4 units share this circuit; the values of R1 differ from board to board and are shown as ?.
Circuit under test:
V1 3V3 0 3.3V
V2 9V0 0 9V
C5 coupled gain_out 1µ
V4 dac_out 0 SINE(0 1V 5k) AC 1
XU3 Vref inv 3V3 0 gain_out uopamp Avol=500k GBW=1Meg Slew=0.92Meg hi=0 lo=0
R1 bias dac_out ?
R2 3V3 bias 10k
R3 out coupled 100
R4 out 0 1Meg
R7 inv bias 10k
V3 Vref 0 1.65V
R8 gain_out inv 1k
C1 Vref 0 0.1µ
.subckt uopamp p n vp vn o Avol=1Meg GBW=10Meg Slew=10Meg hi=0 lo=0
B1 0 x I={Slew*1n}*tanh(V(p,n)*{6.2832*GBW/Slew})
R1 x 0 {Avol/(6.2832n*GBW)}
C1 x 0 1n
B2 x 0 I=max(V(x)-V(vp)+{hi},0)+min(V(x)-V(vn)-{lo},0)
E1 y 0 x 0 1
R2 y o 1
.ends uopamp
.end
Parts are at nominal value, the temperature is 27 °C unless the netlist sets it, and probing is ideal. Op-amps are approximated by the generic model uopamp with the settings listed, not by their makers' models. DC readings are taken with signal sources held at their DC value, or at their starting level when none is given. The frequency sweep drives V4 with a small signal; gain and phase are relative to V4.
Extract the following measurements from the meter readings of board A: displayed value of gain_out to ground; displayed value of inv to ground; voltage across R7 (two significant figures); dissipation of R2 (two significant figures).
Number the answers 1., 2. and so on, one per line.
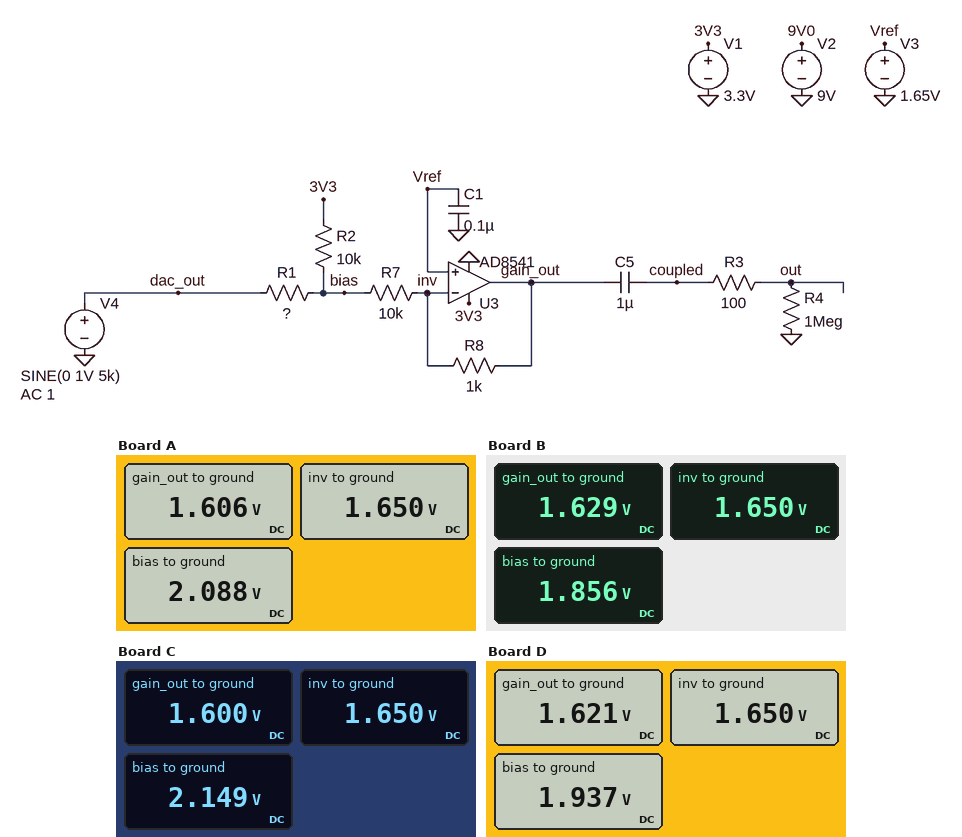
1. 1.606 V
2. 1.650 V
3. 440 mV
4. 150 µW
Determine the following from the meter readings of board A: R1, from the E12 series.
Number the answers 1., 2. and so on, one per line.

1. 27 kΩ
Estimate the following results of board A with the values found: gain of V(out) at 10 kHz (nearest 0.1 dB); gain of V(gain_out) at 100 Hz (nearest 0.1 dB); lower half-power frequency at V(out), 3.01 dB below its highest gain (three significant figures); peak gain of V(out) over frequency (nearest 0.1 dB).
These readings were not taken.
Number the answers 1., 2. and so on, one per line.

1. -36.1 dB
2. -36.1 dB
3. 159 mHz
4. -36.1 dB
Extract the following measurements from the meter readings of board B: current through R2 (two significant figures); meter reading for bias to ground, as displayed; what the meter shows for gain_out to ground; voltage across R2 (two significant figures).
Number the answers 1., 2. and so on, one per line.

1. 140 µA
2. 1.856 V
3. 1.629 V
4. 1.4 V
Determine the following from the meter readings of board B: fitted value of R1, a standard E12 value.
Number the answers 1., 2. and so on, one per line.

1. 15 kΩ
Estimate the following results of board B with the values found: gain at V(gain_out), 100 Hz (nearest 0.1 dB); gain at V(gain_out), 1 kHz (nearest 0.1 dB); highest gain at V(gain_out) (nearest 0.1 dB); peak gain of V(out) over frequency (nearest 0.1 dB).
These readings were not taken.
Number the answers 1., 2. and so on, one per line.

1. -32.0 dB
2. -32.0 dB
3. -32.0 dB
4. -32.0 dB
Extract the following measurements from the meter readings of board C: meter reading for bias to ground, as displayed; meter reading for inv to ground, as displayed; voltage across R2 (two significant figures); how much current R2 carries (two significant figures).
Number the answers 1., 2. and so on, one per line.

1. 2.149 V
2. 1.650 V
3. 1.2 V
4. 120 µA
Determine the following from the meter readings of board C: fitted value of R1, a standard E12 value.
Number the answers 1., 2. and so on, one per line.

1. 33 kΩ
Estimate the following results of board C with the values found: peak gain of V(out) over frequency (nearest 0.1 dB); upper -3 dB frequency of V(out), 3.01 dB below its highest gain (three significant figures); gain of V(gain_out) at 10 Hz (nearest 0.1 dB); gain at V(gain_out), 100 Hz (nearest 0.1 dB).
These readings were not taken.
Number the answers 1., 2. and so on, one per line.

1. -37.6 dB
2. 946 kHz
3. -37.6 dB
4. -37.6 dB
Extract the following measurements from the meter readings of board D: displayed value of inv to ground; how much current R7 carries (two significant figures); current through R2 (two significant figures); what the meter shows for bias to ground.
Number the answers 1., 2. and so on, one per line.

1. 1.650 V
2. 29 µA
3. 140 µA
4. 1.937 V
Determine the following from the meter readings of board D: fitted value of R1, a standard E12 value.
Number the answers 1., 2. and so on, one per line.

1. 18 kΩ
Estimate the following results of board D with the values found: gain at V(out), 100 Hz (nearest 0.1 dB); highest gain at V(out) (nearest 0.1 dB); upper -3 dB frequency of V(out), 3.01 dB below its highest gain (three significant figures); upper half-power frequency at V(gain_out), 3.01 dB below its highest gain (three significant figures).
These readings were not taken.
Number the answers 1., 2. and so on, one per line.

1. -33.3 dB
2. -33.3 dB
3. 943 kHz
4. 943 kHz
